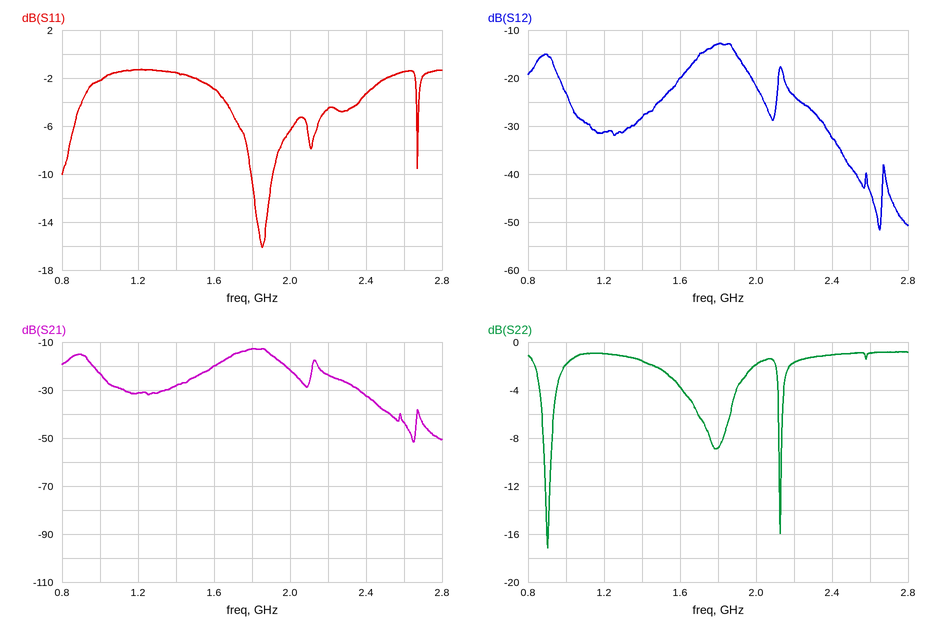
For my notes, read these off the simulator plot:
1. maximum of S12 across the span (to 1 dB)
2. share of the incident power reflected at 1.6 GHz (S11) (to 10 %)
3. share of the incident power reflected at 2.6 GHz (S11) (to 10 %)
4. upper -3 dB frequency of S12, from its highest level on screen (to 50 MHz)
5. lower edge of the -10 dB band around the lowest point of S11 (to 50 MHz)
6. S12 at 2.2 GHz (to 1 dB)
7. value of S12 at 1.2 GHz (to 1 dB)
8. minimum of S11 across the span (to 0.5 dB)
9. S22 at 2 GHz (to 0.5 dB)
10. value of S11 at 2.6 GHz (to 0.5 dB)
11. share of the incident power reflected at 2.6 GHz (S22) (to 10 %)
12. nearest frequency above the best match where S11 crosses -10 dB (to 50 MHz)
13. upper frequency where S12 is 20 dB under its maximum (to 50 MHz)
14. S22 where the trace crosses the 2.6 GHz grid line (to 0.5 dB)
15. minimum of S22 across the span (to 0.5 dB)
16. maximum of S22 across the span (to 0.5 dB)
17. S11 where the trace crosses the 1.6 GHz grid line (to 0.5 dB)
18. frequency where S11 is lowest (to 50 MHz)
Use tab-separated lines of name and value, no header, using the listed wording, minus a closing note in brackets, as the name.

maximum of S12 across the span	-13 dB
share of the incident power reflected at 1.6 GHz (S11)	50 %
share of the incident power reflected at 2.6 GHz (S11)	70 %
upper -3 dB frequency of S12, from its highest level on screen	1.90 GHz
lower edge of the -10 dB band around the lowest point of S11	1.80 GHz
S12 at 2.2 GHz	-24 dB
value of S12 at 1.2 GHz	-31 dB
minimum of S11 across the span	-16.0 dB
S22 at 2 GHz	-2.0 dB
value of S11 at 2.6 GHz	-1.5 dB
share of the incident power reflected at 2.6 GHz (S22)	80 %
nearest frequency above the best match where S11 crosses -10 dB	1.90 GHz
upper frequency where S12 is 20 dB under its maximum	2.40 GHz
S22 where the trace crosses the 2.6 GHz grid line	-1.0 dB
minimum of S22 across the span	-17.0 dB
maximum of S22 across the span	-1.0 dB
S11 where the trace crosses the 1.6 GHz grid line	-3.0 dB
frequency where S11 is lowest	1.85 GHz
